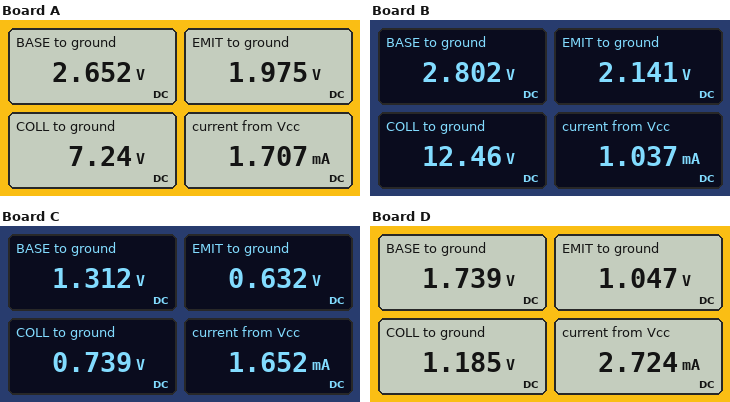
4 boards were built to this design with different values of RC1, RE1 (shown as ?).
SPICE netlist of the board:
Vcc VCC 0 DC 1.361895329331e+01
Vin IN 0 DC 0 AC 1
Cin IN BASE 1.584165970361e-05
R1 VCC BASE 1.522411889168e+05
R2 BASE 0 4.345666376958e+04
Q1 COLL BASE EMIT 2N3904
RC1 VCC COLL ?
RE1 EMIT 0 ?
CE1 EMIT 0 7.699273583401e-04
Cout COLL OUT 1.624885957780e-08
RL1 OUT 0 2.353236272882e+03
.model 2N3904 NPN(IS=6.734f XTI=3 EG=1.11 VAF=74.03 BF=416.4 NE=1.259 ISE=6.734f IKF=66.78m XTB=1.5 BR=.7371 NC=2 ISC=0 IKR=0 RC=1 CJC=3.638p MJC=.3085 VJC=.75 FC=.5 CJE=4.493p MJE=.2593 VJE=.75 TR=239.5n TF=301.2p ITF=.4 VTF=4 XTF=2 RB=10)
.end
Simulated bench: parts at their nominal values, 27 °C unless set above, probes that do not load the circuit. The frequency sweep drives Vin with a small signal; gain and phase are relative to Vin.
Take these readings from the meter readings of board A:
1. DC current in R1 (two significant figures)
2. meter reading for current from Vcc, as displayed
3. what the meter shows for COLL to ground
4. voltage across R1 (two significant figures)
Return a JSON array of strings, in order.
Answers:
["72 µA", "1.707 mA", "7.24 V", "11 V"]
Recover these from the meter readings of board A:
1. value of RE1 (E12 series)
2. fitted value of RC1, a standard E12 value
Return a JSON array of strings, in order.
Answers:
["1.2 kΩ", "3.9 kΩ"]
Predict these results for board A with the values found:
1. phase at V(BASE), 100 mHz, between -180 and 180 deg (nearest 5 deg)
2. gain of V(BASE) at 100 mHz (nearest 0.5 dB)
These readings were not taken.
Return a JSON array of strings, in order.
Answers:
["70 deg", "-11.5 dB"]
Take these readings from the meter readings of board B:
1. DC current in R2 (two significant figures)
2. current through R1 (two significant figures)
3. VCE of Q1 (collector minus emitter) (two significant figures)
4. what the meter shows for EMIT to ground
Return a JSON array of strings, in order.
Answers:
["64 µA", "71 µA", "10 V", "2.141 V"]
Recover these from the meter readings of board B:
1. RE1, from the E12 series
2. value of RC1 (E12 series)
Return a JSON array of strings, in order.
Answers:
["2.2 kΩ", "1.2 kΩ"]
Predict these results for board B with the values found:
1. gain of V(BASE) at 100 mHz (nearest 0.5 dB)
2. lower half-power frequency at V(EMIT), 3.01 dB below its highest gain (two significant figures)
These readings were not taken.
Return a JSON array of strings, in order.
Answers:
["-11.0 dB", "240 mHz"]
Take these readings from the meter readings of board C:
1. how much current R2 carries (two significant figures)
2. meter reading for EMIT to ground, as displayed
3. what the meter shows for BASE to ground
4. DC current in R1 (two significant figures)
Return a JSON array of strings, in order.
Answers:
["30 µA", "0.632 V", "1.312 V", "81 µA"]
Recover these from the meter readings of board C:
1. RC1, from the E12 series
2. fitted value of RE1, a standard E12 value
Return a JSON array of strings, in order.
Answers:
["8.2 kΩ", "390 Ω"]
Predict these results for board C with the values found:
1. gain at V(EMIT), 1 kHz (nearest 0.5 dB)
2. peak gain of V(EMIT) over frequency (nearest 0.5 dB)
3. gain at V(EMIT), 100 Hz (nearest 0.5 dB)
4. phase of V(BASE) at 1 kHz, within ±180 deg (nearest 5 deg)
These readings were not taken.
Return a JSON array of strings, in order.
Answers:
["-45.0 dB", "-33.5 dB", "-34.0 dB", "15 deg"]
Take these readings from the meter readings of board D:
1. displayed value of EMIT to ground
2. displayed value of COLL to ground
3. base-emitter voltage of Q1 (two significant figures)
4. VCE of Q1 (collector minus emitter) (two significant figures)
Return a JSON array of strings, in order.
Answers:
["1.047 V", "1.185 V", "690 mV", "140 mV"]
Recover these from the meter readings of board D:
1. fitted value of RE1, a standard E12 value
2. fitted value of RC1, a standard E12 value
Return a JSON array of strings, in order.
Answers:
["390 Ω", "4.7 kΩ"]
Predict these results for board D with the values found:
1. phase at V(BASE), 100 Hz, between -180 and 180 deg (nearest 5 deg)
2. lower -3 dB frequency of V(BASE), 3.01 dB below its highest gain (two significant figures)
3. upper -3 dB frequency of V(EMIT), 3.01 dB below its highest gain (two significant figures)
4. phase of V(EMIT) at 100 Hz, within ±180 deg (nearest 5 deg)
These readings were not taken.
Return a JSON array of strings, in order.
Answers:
["70 deg", "340 Hz", "350 Hz", "-15 deg"]
